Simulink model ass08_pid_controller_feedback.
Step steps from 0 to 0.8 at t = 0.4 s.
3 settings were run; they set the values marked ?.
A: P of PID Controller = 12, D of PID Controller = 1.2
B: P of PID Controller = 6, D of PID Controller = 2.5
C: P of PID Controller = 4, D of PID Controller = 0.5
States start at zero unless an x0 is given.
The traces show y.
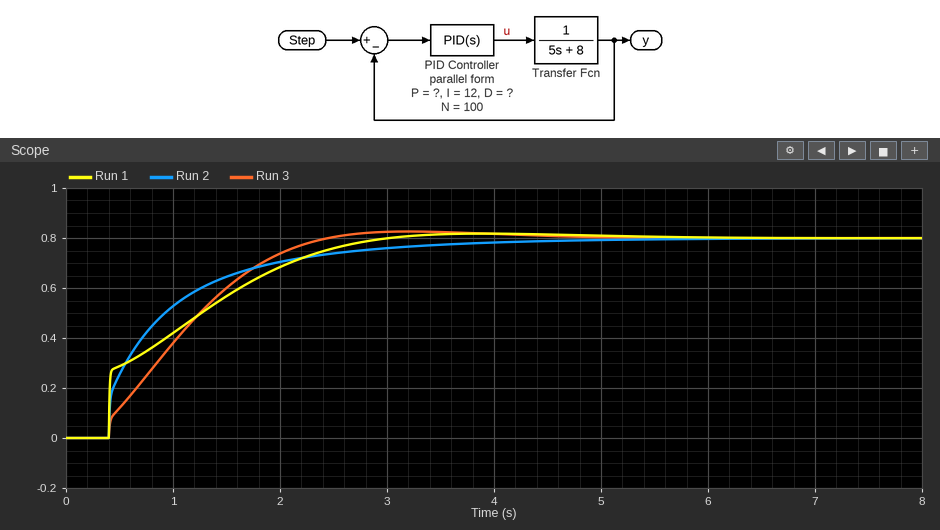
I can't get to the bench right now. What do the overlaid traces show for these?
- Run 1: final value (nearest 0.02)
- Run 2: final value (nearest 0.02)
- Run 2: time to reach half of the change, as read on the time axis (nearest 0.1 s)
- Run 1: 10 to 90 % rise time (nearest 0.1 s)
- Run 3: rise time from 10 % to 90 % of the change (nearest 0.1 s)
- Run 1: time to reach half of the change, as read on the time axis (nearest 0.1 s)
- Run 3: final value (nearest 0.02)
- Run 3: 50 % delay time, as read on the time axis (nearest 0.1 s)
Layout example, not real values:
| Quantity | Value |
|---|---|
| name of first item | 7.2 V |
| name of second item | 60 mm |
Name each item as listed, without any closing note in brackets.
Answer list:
| Quantity | Value |
|---|---|
| Run 1: final value | 0.80 |
| Run 2: final value | 0.80 |
| Run 2: time to reach half of the change, as read on the time axis | 0.7 s |
| Run 1: 10 to 90 % rise time | 1.8 s |
| Run 3: rise time from 10 % to 90 % of the change | 1.5 s |
| Run 1: time to reach half of the change, as read on the time axis | 0.9 s |
| Run 3: final value | 0.80 |
| Run 3: 50 % delay time, as read on the time axis | 1.0 s |
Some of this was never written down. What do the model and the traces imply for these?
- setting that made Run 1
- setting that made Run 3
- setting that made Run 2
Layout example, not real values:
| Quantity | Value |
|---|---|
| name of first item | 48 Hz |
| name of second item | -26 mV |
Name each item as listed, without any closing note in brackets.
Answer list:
| Quantity | Value |
|---|---|
| setting that made Run 1 | B |
| setting that made Run 3 | C |
| setting that made Run 2 | A |
